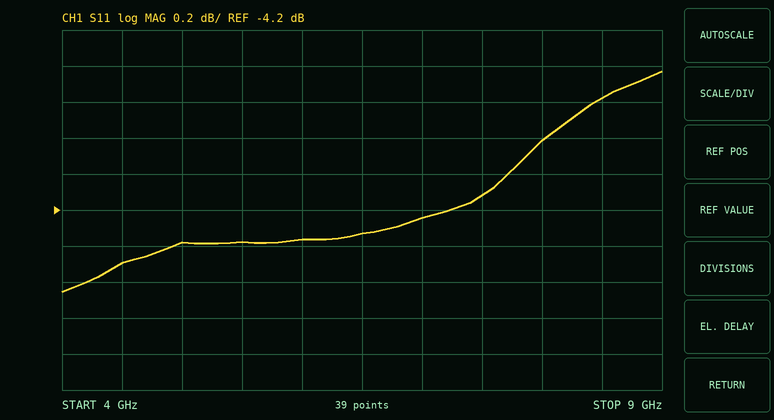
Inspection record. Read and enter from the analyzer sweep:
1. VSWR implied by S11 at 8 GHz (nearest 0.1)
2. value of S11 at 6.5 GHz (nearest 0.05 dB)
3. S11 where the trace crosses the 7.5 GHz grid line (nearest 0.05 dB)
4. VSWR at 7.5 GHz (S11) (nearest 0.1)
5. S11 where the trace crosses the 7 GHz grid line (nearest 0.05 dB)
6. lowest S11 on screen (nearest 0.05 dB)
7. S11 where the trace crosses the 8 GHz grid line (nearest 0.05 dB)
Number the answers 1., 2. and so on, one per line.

1. 4.6
2. -4.35 dB
3. -4.10 dB
4. 4.3
5. -4.25 dB
6. -4.65 dB
7. -3.80 dB
